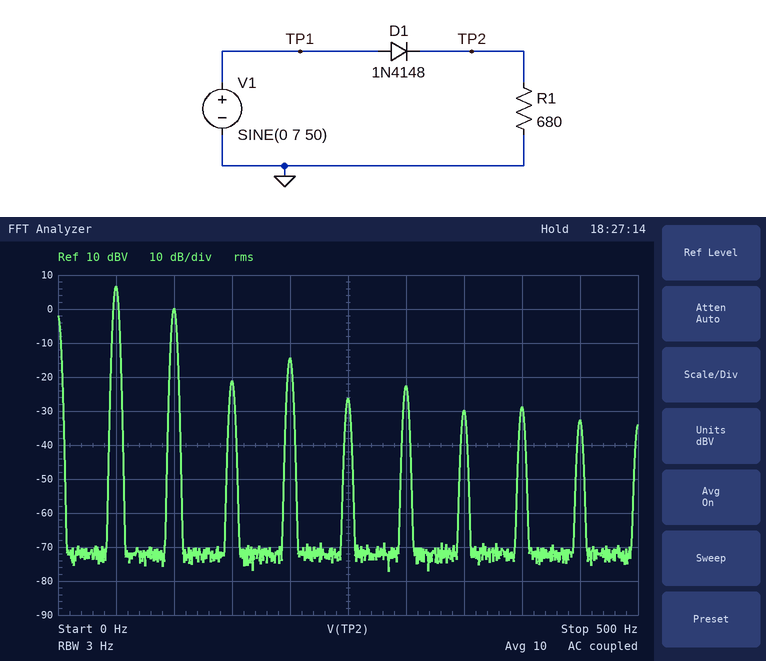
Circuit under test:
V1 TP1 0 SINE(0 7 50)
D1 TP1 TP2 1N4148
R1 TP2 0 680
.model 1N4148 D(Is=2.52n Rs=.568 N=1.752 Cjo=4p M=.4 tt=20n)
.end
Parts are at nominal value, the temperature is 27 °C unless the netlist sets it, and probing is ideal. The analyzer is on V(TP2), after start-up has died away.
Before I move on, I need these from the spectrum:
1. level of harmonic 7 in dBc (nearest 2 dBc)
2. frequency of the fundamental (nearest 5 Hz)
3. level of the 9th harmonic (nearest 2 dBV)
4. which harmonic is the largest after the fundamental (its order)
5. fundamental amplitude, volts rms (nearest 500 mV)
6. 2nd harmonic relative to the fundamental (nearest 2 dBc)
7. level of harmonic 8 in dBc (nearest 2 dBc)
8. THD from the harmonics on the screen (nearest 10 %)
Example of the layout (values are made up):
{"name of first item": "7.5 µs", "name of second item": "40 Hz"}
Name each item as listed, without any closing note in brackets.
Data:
{"level of harmonic 7 in dBc": "-36 dBc", "frequency of the fundamental": "50 Hz", "level of the 9th harmonic": "-32 dBV", "which harmonic is the largest after the fundamental": "2", "fundamental amplitude, volts rms": "2.0 V", "2nd harmonic relative to the fundamental": "-6 dBc", "level of harmonic 8 in dBc": "-36 dBc", "THD from the harmonics on the screen": "50 %"}
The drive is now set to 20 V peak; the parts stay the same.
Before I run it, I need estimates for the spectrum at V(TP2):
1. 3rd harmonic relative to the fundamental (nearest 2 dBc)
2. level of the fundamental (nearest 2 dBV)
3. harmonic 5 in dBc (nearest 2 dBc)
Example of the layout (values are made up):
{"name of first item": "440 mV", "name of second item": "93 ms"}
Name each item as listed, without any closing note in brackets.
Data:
{"3rd harmonic relative to the fundamental": "-36 dBc", "level of the fundamental": "16 dBV", "harmonic 5 in dBc": "-42 dBc"}
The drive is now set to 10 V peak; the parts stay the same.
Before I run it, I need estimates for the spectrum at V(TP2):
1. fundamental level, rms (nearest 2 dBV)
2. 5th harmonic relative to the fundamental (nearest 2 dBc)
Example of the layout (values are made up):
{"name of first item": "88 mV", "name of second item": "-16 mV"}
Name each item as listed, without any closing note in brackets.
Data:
{"fundamental level, rms": "10 dBV", "5th harmonic relative to the fundamental": "-36 dBc"}
